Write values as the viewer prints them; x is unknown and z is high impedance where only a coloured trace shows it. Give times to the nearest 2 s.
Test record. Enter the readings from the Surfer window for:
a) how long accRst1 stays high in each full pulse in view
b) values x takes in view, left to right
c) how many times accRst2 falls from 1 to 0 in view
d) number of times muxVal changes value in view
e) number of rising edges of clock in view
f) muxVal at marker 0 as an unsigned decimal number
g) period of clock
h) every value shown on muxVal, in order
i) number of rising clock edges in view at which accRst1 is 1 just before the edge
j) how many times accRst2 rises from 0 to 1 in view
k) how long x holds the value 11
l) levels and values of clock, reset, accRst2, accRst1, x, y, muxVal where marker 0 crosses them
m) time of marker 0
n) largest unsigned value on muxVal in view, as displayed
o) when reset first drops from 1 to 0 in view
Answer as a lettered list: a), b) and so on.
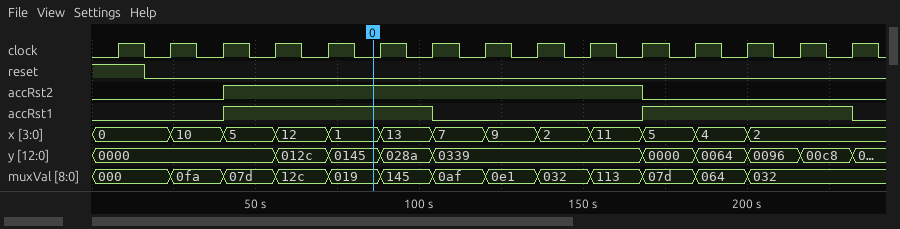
a) 64 s, 64 s
b) 0, 10, 5, 12, 1, 13, 7, 9, 2, 11, 5, 4, 2
c) 1
d) 12
e) 15
f) 25
g) 16 s
h) 000, 0fa, 07d, 12c, 019, 145, 0af, 0e1, 032, 113, 07d, 064, 032
i) 8
j) 1
k) 16 s
l) clock=0, reset=0, accRst2=1, accRst1=1, x=1, y=0145, muxVal=019
m) 86 s
n) 145
o) 16 s
